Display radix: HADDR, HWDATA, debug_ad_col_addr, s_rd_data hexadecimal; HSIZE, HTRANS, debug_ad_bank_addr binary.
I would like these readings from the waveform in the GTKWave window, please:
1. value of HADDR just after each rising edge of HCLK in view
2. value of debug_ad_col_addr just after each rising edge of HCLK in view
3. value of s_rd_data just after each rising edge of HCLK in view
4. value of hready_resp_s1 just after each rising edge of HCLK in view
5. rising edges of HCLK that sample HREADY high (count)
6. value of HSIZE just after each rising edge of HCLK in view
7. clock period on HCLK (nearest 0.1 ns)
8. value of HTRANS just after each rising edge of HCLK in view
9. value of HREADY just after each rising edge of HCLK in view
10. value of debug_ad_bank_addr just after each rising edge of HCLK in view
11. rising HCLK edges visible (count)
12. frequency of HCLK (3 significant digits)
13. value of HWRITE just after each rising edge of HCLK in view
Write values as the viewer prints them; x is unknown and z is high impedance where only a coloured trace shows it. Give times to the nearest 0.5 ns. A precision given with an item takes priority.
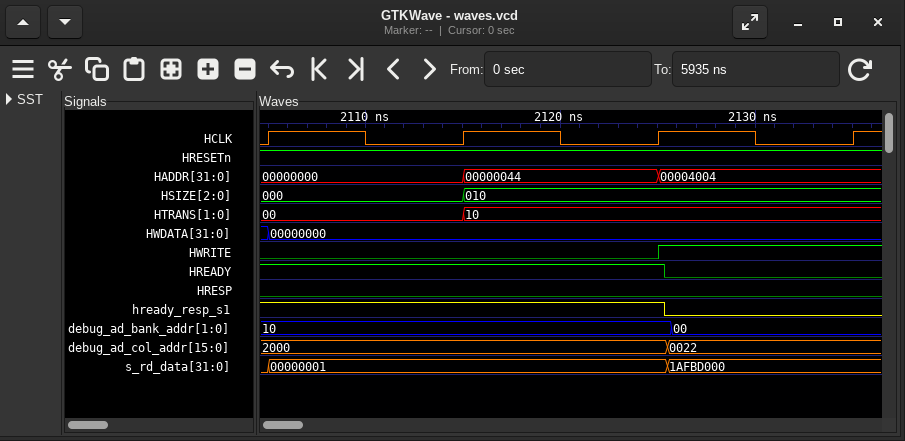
00000000, 00000044, 00004004, 00004004
2000, 2000, 2000, 0022
00000001, 00000001, 00000001, 1AFBD000
1 1 1 0
3
000, 010, 010, 010
10 ns
00, 10, 10, 10
1 1 1 0
10, 10, 10, 00
4
100 MHz
0 0 1 1
